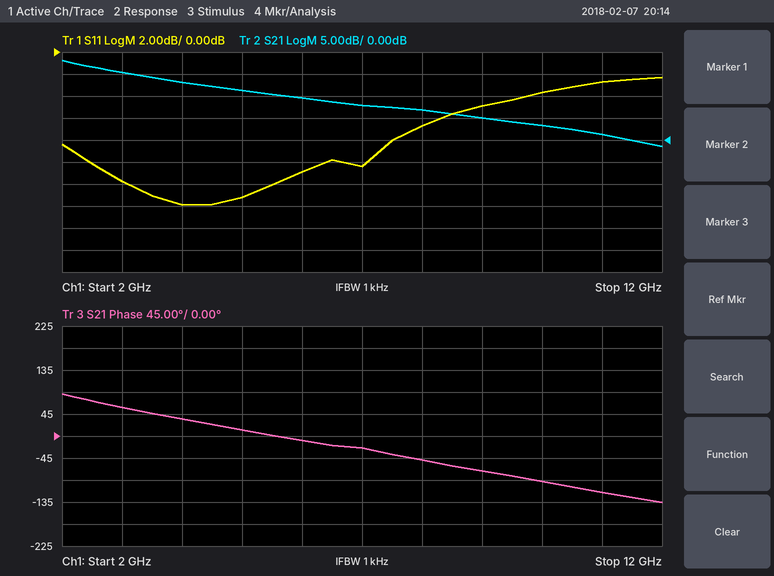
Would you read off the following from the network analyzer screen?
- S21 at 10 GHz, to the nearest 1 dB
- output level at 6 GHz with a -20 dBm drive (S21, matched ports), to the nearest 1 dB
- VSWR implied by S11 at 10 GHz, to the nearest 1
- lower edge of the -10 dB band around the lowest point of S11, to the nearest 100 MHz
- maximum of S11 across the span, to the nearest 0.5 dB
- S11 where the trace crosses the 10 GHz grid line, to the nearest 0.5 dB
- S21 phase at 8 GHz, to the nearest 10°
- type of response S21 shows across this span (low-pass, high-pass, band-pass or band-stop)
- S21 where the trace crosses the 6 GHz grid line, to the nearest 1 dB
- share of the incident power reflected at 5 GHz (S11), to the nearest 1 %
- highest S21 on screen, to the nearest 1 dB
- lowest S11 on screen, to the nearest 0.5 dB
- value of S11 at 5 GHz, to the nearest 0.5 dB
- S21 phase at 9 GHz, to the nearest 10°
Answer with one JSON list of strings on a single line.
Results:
["3 dB", "-10 dBm", "5", "2.5 GHz", "-2.5 dB", "-3.5 dB", "-50°", "low-pass", "10 dB", "5 %", "18 dB", "-14.0 dB", "-13.0 dB", "-70°"]
